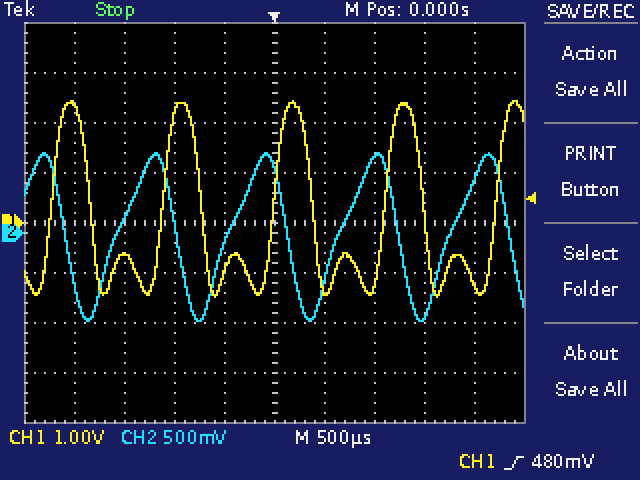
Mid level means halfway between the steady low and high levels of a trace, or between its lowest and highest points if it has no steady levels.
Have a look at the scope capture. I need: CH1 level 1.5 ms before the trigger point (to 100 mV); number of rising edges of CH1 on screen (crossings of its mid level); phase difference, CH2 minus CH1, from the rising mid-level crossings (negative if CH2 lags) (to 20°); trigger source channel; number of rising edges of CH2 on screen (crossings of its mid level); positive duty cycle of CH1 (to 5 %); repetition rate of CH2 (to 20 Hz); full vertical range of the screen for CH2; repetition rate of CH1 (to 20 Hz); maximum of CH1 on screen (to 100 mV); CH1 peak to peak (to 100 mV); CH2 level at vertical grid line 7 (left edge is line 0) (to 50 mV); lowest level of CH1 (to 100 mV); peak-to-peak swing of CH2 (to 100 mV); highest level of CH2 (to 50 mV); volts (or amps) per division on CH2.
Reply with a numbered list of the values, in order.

1. -600 mV
2. 5
3. +160°
4. CH1
5. 4
6. 35 %
7. 900 Hz
8. 4 V
9. 900 Hz
10. 2.4 V
11. 3.9 V
12. 750 mV
13. -1.5 V
14. 1.70 V
15. 800 mV
16. 500 mV
